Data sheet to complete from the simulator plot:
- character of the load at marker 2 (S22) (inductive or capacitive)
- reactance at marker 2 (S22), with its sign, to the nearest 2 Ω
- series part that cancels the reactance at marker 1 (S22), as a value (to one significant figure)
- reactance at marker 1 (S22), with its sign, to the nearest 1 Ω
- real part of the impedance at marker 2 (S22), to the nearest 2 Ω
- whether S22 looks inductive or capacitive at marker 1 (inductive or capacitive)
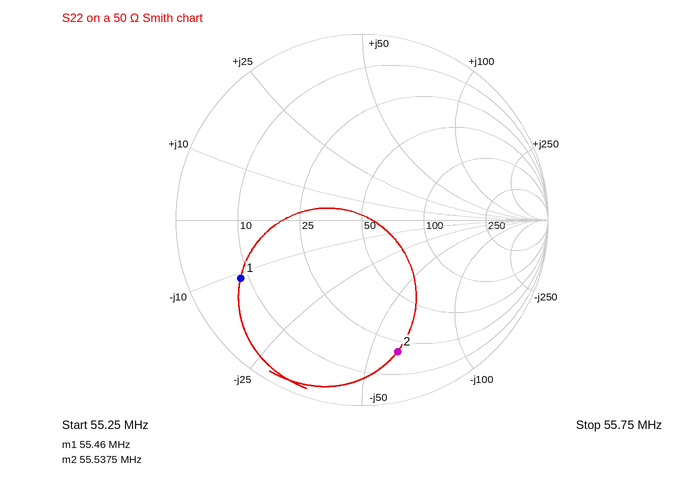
capacitive
-62 Ω
30 nH
-11 Ω
20 Ω
capacitive
